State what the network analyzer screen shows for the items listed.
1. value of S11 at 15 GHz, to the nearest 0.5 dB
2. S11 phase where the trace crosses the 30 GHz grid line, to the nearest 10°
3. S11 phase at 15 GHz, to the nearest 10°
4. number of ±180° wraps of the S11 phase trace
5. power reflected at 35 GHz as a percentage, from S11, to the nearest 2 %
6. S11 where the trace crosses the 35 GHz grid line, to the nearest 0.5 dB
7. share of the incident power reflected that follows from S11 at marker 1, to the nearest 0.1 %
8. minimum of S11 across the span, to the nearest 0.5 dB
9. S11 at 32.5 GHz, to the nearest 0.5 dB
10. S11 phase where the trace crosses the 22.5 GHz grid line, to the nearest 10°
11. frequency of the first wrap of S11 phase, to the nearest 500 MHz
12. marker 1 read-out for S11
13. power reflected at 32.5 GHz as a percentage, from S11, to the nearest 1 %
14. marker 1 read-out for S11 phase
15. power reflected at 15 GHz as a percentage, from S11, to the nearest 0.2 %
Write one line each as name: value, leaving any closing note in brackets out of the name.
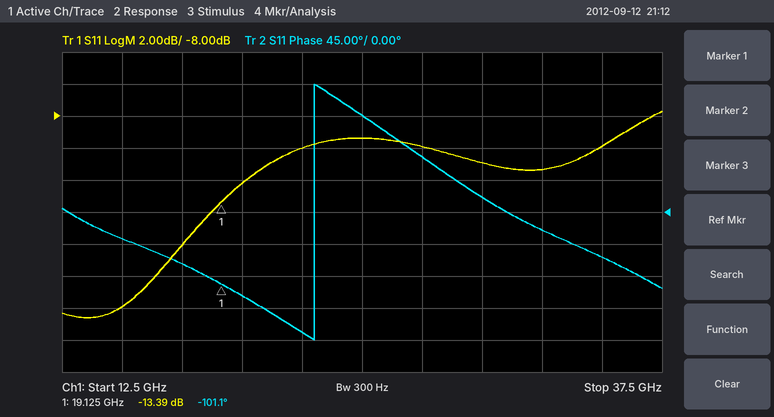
value of S11 at 15 GHz, to the nearest 0.5 dB: -20.0 dB
S11 phase where the trace crosses the 30 GHz grid line, to the nearest 10°: 20°
S11 phase at 15 GHz, to the nearest 10°: -40°
number of ±180° wraps of the S11 phase trace: 1
power reflected at 35 GHz as a percentage, from S11, to the nearest 2 %: 10 %
S11 where the trace crosses the 35 GHz grid line, to the nearest 0.5 dB: -10.0 dB
share of the incident power reflected that follows from S11 at marker 1, to the nearest 0.1 %: 4.6 %
minimum of S11 across the span, to the nearest 0.5 dB: -20.5 dB
S11 at 32.5 GHz, to the nearest 0.5 dB: -11.5 dB
S11 phase where the trace crosses the 22.5 GHz grid line, to the nearest 10°: -170°
frequency of the first wrap of S11 phase, to the nearest 500 MHz: 23.0 GHz
marker 1 read-out for S11: -13.39 dB
power reflected at 32.5 GHz as a percentage, from S11, to the nearest 1 %: 7 %
marker 1 read-out for S11 phase: -101.1°
power reflected at 15 GHz as a percentage, from S11, to the nearest 0.2 %: 1.0 %
